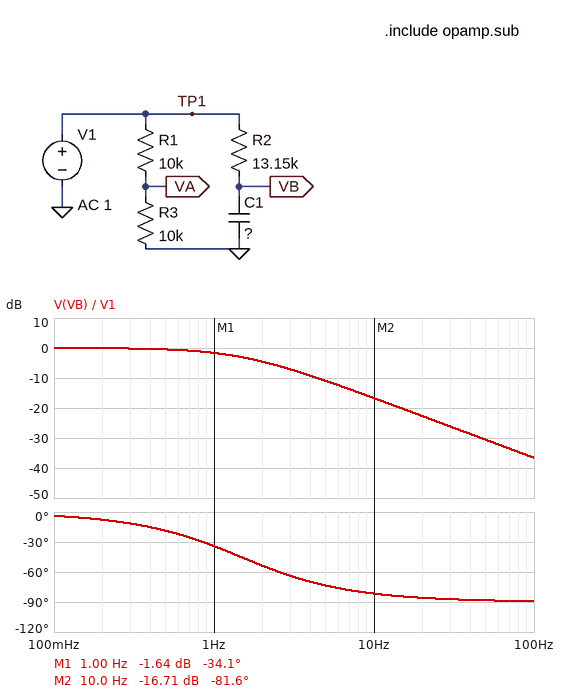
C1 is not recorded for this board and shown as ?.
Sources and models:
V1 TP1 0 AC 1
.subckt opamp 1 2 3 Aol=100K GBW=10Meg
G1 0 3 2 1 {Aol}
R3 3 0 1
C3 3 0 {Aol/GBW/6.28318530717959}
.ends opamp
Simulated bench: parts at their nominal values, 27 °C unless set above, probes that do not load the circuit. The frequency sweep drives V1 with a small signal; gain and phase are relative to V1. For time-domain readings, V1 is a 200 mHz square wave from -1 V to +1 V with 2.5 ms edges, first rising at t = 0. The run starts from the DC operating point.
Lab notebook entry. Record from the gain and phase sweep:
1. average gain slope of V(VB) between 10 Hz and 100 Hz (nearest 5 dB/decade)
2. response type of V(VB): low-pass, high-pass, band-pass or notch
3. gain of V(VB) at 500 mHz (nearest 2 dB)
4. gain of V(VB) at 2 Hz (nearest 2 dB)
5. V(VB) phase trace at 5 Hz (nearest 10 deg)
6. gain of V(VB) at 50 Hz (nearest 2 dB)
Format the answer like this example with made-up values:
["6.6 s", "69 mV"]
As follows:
["-20 dB/decade", "low-pass", "0 dB", "-4 dB", "-70 deg", "-30 dB"]
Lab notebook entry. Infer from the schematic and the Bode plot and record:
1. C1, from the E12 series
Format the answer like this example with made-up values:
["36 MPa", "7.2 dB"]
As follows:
["8.2 µF"]
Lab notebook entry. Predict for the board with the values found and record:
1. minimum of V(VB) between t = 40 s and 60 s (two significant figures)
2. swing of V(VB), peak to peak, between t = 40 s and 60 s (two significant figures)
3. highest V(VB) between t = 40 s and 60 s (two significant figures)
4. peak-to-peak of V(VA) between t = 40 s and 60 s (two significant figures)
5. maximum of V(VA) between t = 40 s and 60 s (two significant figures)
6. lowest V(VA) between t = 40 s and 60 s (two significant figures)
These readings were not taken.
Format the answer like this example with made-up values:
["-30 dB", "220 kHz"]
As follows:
["-1.0 V", "2.0 V", "1.0 V", "1.0 V", "500 mV", "-500 mV"]
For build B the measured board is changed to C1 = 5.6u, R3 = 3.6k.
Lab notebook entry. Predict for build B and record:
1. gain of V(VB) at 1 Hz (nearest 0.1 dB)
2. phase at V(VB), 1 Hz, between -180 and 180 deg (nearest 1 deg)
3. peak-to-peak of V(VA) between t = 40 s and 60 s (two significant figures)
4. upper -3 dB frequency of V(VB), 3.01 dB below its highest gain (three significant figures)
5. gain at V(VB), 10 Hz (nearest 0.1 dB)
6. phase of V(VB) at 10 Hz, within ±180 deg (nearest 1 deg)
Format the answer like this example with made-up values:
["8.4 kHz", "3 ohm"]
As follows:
["-0.8 dB", "-25 deg", "530 mV", "2.16 Hz", "-13.5 dB", "-78 deg"]
